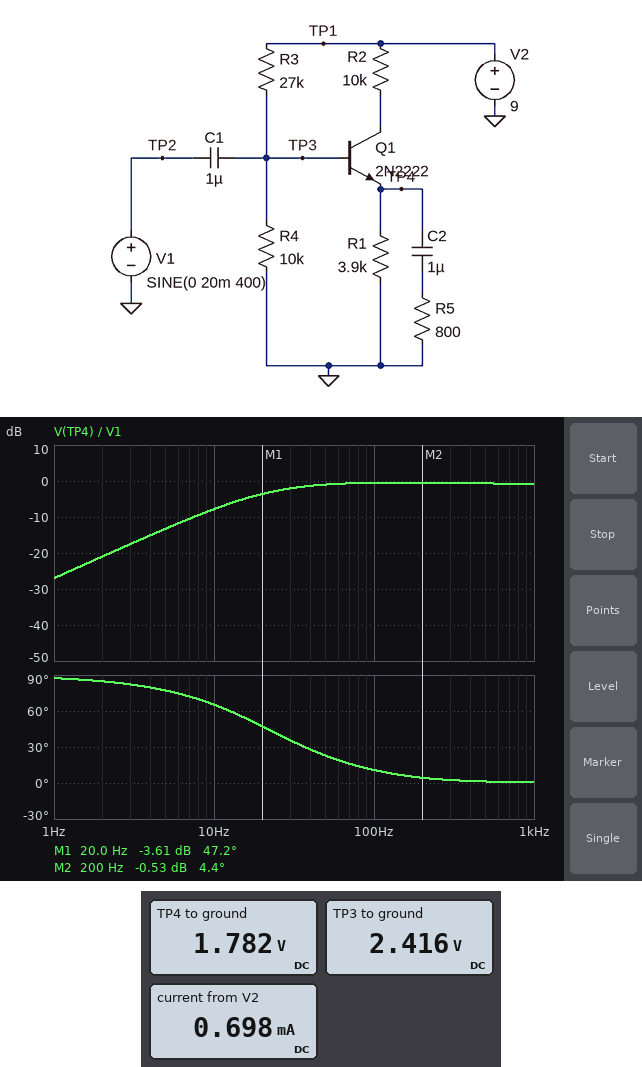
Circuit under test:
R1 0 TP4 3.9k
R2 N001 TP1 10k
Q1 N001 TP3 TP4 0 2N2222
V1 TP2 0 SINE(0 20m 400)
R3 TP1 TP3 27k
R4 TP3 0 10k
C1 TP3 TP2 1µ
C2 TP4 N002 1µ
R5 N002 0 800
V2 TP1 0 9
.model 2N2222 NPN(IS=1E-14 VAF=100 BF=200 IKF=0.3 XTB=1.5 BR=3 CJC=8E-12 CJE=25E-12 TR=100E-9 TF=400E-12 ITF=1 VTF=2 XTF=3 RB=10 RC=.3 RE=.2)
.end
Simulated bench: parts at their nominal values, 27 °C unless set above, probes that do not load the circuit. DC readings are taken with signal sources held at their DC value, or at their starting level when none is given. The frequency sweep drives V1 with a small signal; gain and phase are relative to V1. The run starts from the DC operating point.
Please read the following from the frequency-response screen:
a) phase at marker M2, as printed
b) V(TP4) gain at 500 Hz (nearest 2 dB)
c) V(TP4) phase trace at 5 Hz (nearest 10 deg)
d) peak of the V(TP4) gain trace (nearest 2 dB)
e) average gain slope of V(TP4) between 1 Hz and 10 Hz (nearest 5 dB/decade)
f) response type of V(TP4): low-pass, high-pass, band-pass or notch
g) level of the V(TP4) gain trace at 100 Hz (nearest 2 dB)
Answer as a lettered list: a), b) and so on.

a) 4.4 deg
b) 0 dB
c) 80 deg
d) 0 dB
e) 20 dB/decade
f) high-pass
g) 0 dB
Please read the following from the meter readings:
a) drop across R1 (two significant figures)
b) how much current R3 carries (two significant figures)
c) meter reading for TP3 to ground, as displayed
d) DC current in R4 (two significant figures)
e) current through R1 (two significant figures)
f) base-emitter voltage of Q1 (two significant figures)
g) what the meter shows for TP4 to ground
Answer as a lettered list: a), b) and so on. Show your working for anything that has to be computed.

a) 1.782 V = 1.8 V
b) (9 V - 2.416 V) / 27 kΩ = 240 µA
c) 2.416 V
d) (2.416 V) / 10 kΩ = 240 µA
e) (1.782 V) / 3.9 kΩ = 460 µA
f) 2.416 V - 1.782 V = 630 mV
g) 1.782 V
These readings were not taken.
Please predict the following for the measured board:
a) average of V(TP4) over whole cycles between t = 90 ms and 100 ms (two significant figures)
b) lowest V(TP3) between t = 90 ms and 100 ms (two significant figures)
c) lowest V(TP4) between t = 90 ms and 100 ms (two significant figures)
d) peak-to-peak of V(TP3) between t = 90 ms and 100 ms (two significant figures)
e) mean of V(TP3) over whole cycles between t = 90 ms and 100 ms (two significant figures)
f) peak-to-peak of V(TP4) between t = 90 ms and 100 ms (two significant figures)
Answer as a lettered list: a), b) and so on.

a) 1.8 V
b) 2.4 V
c) 1.8 V
d) 40 mV
e) 2.4 V
f) 37 mV
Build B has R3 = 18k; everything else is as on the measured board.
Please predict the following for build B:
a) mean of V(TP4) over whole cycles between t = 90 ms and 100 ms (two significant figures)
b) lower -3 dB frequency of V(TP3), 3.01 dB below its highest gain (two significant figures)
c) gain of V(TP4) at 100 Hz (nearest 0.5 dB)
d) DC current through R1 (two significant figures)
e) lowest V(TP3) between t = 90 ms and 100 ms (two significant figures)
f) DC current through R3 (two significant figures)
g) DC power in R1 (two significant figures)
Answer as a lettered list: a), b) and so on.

a) 2.5 V
b) 190 Hz
c) -5.0 dB
d) 650 µA
e) 3.1 V
f) 320 µA
g) 1.6 mW
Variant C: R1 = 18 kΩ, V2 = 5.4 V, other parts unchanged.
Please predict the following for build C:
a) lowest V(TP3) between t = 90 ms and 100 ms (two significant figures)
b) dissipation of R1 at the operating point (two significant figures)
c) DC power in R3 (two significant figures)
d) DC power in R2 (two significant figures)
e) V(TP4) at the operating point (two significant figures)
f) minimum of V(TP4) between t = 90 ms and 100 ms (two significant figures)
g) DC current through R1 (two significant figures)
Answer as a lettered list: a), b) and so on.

a) 1.4 V
b) 43 µW
c) 580 µW
d) 24 µW
e) 880 mV
f) 870 mV
g) 49 µA
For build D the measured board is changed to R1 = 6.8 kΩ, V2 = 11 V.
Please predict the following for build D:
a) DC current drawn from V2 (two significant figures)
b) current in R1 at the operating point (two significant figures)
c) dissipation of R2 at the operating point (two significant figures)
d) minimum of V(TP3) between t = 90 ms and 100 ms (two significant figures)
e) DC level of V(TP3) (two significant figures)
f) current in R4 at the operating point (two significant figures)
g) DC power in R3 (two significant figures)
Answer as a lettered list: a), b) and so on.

a) 640 µA
b) 340 µA
c) 1.2 mW
d) 2.9 V
e) 3.0 V
f) 300 µA
g) 2.4 mW
